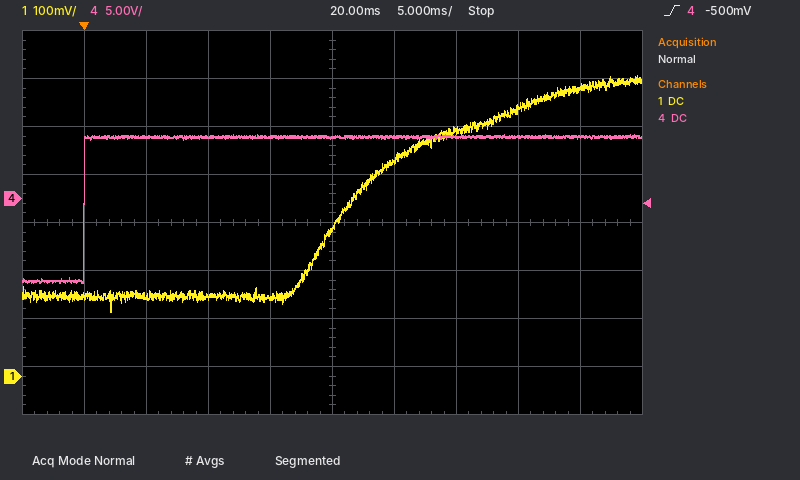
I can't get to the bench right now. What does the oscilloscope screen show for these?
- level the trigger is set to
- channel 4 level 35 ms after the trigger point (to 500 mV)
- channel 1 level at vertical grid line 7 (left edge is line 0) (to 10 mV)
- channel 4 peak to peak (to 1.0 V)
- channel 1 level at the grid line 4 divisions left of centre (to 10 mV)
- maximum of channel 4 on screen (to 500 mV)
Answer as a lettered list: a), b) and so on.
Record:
a) -500 mV
b) 6.5 V
c) 510 mV
d) 15.0 V
e) 170 mV
f) 6.5 V
